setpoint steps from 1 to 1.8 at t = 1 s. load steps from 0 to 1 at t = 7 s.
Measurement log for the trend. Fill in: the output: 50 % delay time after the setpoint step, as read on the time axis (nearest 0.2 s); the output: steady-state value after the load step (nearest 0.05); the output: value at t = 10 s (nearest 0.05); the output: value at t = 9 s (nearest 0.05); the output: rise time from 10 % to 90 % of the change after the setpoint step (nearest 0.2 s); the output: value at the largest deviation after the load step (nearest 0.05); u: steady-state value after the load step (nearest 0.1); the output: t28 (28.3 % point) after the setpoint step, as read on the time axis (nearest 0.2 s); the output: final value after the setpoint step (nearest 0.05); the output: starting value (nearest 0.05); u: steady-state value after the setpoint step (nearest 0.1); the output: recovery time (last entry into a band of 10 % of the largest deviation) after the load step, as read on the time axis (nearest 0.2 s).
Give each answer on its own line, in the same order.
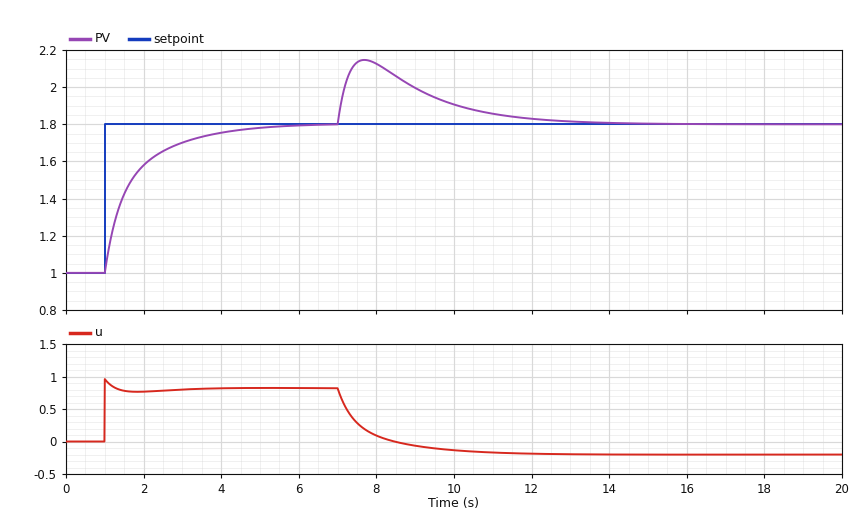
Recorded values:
1.4 s
1.80
1.90
2.00
2.2 s
2.15
-0.2
1.2 s
1.80
1.00
0.8
11.8 s
